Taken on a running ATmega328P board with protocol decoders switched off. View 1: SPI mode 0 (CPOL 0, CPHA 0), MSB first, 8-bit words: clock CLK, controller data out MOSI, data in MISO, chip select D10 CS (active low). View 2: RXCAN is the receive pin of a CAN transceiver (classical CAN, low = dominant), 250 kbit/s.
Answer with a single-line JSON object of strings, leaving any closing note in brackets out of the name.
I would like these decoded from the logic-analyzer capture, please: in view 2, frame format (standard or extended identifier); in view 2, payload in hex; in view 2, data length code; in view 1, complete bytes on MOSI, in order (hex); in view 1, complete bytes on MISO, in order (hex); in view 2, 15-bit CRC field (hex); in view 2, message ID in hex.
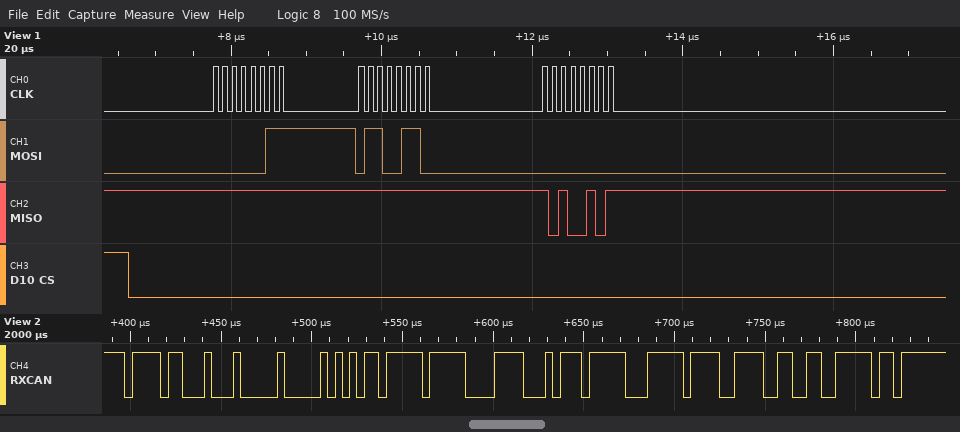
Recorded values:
{"in view 2, frame format": "standard", "in view 2, payload in hex": "00 AD FF 8F 17 7C FF 9E", "in view 2, data length code": "8", "in view 1, complete bytes on MOSI, in order": "03 66 00", "in view 1, complete bytes on MISO, in order": "FF FF A5", "in view 2, 15-bit CRC field": "0x333F", "in view 2, message ID in hex": "0x7B1"}
